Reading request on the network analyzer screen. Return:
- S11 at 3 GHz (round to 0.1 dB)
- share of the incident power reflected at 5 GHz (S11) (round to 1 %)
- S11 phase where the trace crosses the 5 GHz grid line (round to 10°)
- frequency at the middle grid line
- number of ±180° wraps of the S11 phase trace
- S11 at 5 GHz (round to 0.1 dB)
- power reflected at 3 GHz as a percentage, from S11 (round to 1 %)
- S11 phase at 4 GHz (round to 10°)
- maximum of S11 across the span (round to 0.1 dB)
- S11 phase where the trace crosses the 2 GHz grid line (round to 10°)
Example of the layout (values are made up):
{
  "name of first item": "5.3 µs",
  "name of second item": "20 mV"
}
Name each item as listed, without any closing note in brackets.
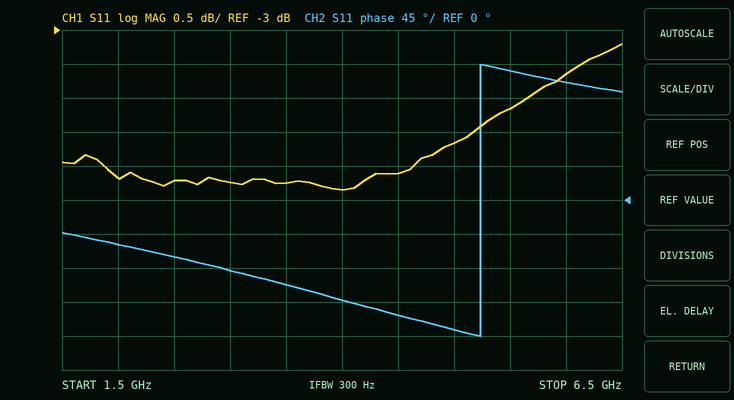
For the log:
{
  "S11 at 3 GHz": "-5.2 dB",
  "share of the incident power reflected at 5 GHz (S11)": "34 %",
  "S11 phase where the trace crosses the 5 GHz grid line": "-170°",
  "frequency at the middle grid line": "4 GHz",
  "number of ±180° wraps of the S11 phase trace": "1",
  "S11 at 5 GHz": "-4.7 dB",
  "power reflected at 3 GHz as a percentage, from S11": "30 %",
  "S11 phase at 4 GHz": "-130°",
  "maximum of S11 across the span": "-3.2 dB",
  "S11 phase where the trace crosses the 2 GHz grid line": "-60°"
}
